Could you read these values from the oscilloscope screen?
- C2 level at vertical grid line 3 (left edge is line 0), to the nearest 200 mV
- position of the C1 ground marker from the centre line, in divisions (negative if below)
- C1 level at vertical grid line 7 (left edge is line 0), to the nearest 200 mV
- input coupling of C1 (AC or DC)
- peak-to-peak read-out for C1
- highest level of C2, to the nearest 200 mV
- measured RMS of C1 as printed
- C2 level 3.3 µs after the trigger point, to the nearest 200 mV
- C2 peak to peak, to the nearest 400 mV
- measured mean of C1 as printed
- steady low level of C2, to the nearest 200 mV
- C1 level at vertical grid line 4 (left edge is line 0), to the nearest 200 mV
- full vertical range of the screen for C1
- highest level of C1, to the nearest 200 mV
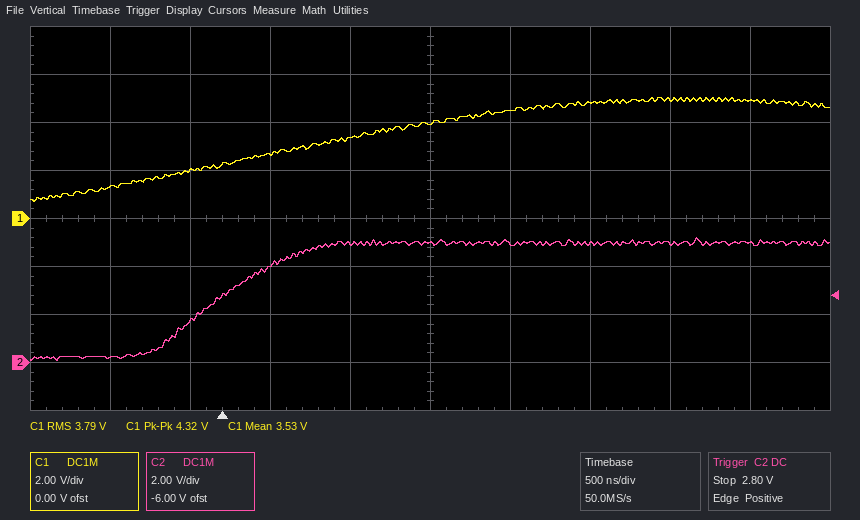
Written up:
4.0 V
0.0 div
4.8 V
DC
4.32 V
5.2 V
3.79 V
5.0 V
5.2 V
3.53 V
200 mV
3.4 V
16 V
5.0 V
